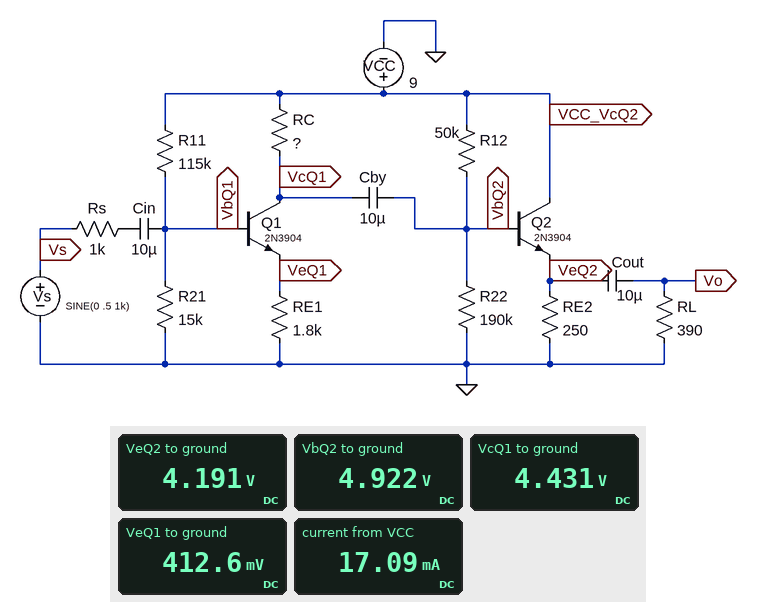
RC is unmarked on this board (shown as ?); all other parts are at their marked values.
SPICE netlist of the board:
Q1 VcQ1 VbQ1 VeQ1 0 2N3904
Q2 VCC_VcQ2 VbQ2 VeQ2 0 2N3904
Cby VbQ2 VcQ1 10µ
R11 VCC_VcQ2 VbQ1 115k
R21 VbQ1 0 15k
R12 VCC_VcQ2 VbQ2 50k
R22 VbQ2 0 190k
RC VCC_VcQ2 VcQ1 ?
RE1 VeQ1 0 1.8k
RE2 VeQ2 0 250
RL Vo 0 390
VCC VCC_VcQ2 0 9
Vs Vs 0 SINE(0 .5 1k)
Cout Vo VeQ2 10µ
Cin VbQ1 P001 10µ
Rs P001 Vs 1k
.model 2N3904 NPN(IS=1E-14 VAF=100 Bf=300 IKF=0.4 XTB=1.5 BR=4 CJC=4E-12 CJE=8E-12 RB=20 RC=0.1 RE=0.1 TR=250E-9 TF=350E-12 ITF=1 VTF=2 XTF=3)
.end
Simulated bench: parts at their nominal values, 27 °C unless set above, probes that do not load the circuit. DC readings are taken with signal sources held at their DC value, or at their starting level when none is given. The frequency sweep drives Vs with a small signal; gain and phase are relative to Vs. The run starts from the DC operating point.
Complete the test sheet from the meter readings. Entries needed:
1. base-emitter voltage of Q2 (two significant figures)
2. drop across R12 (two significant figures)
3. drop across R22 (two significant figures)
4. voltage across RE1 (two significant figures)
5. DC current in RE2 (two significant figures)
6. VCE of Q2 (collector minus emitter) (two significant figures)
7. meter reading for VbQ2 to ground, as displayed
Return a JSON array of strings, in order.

["730 mV", "4.1 V", "4.9 V", "410 mV", "17 mA", "4.8 V", "4.922 V"]
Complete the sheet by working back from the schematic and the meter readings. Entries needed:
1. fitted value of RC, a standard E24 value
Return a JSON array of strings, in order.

["20 kΩ"]
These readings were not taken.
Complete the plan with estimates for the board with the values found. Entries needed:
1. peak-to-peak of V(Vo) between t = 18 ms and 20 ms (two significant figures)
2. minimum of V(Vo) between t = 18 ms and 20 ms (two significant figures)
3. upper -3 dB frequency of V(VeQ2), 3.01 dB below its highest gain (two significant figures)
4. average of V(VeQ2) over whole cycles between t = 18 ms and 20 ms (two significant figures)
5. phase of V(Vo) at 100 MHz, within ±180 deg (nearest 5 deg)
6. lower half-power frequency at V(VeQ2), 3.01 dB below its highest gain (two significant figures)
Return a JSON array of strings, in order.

["4.6 V", "-2.4 V", "1.6 MHz", "4.1 V", "-25 deg", "1.2 Hz"]
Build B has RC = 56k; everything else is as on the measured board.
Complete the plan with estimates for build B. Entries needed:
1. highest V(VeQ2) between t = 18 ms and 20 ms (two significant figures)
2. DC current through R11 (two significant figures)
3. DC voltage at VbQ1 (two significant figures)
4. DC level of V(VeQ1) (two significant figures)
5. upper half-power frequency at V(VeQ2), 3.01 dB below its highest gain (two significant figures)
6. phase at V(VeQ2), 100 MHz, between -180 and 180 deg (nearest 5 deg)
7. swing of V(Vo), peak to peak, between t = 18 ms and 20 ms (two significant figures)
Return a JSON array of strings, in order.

["6.6 V", "70 µA", "910 mV", "300 mV", "52 MHz", "-55 deg", "2.5 V"]
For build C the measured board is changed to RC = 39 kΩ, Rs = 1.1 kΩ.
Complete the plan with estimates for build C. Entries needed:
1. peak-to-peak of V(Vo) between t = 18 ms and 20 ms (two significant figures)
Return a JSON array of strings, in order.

["3.1 V"]
